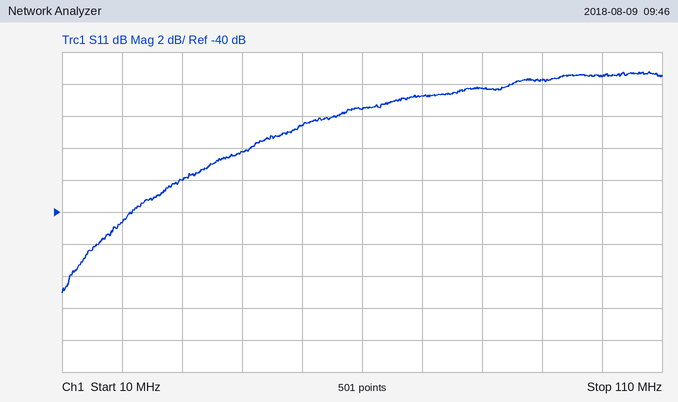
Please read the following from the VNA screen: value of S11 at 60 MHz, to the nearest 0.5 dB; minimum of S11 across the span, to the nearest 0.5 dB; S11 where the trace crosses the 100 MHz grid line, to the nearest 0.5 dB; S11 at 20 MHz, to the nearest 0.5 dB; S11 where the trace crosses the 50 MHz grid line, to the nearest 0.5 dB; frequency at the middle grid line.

-33.5 dB
-45.0 dB
-31.5 dB
-40.5 dB
-34.5 dB
60 MHz
